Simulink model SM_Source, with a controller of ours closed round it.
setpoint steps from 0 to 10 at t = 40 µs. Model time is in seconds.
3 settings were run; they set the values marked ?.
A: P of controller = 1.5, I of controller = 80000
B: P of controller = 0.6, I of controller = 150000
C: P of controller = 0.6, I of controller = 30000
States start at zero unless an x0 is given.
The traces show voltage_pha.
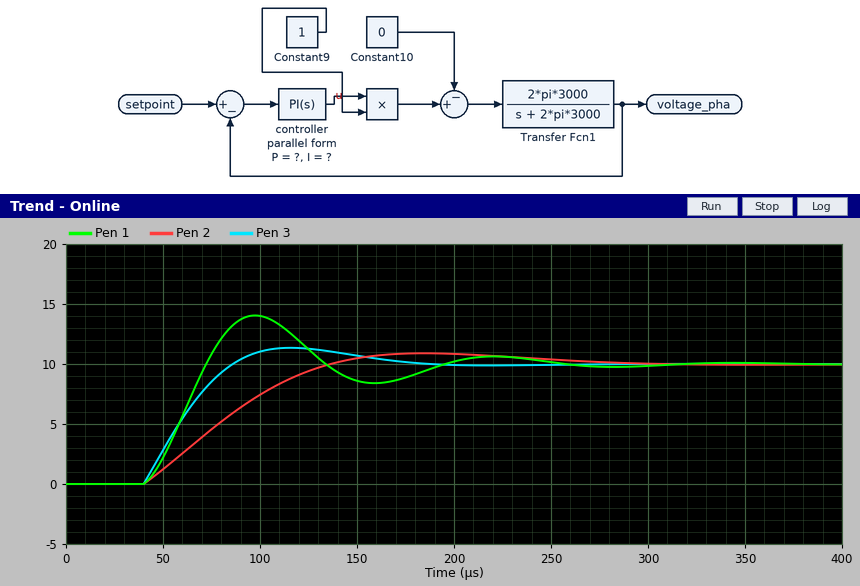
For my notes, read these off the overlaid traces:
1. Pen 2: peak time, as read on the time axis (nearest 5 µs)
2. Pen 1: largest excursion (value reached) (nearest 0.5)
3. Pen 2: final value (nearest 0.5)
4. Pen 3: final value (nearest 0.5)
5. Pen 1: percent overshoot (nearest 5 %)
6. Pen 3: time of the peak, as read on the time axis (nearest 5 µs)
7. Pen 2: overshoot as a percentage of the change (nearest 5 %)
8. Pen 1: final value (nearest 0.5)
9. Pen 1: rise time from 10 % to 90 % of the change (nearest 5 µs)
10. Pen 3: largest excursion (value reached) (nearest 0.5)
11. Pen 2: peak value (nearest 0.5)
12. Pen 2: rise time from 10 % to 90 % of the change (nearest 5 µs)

185 µs
14.0
10.0
10.0
40 %
115 µs
10 %
10.0
25 µs
11.5
11.0
70 µs
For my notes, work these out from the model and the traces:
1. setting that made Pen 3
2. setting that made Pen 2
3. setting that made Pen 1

A
C
B
